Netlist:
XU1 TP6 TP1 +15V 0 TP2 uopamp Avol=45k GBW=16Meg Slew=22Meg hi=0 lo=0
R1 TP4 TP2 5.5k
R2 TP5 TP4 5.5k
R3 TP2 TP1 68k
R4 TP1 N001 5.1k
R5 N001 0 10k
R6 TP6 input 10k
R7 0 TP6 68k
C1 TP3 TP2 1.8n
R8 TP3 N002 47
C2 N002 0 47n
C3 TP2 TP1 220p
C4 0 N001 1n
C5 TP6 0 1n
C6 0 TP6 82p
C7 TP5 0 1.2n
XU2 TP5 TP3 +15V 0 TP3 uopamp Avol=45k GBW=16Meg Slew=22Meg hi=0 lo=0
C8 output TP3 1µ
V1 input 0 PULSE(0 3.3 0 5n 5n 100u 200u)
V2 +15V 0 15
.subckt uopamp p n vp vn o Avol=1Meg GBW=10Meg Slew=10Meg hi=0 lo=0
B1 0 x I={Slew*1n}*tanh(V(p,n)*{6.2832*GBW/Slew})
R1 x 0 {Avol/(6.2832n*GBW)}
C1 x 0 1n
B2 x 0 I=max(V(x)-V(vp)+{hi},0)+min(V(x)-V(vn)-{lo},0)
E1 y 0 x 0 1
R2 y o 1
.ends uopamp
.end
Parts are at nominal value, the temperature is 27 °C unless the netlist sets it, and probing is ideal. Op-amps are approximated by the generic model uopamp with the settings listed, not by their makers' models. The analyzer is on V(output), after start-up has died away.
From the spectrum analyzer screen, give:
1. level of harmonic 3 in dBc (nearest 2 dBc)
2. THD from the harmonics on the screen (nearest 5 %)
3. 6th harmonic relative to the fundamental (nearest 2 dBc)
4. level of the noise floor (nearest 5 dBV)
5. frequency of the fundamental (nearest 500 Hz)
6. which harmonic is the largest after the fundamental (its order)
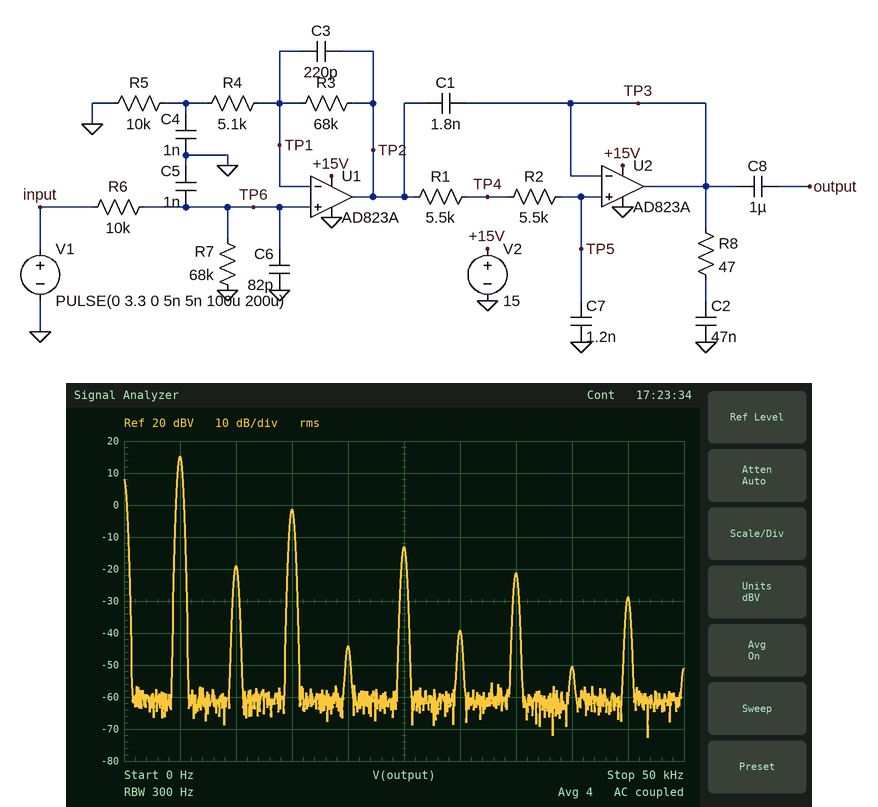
-16 dBc
15 %
-54 dBc
-60 dBV
5.0 kHz
3
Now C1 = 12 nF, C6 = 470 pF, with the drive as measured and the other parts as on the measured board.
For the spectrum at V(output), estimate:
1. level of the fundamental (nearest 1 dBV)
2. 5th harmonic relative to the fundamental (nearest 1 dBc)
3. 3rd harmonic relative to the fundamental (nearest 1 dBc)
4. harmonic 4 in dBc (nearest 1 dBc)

15 dBV
-30 dBc
-18 dBc
-52 dBc
